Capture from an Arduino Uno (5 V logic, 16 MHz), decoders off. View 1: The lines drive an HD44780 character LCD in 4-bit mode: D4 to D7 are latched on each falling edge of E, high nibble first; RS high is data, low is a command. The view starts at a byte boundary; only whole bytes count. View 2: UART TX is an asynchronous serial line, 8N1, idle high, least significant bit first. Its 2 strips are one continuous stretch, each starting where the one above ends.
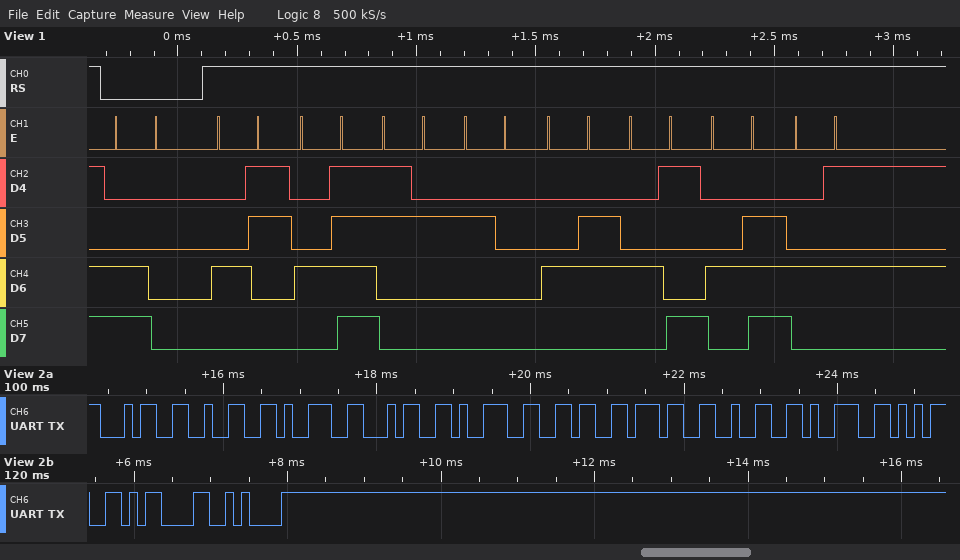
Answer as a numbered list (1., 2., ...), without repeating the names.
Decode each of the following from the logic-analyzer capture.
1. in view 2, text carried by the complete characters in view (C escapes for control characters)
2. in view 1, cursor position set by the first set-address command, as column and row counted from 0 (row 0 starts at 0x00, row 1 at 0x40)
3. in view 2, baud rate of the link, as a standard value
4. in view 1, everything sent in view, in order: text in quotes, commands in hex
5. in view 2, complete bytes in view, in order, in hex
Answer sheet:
1. "4294967295\r\n"
2. column 0, row 1
3. 9600 baud
4. 0xC0 "CO2 FINE"
5. 34 32 39 34 39 36 37 32 39 35 0D 0A
